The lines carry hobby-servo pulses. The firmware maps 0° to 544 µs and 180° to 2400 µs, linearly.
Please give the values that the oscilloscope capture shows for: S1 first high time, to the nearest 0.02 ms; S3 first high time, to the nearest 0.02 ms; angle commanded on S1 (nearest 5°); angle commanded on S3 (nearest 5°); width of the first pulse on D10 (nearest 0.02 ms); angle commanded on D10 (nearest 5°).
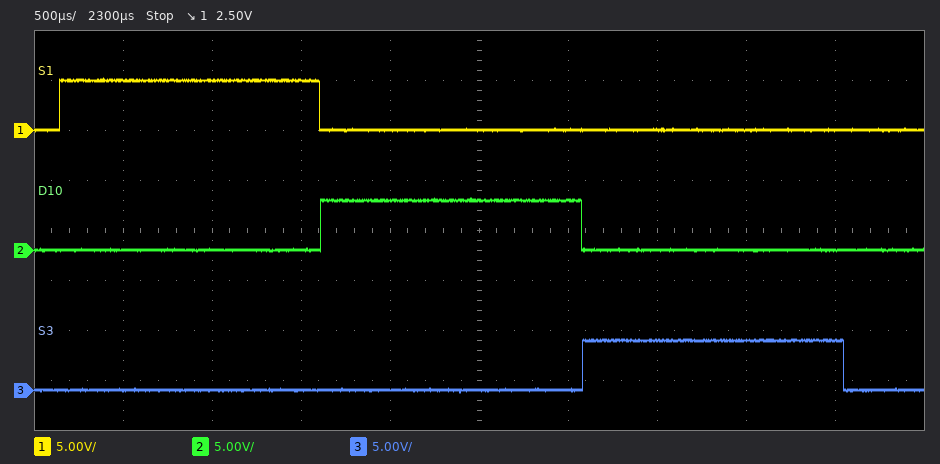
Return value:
1.46 ms
1.46 ms
90°
90°
1.46 ms
90°
